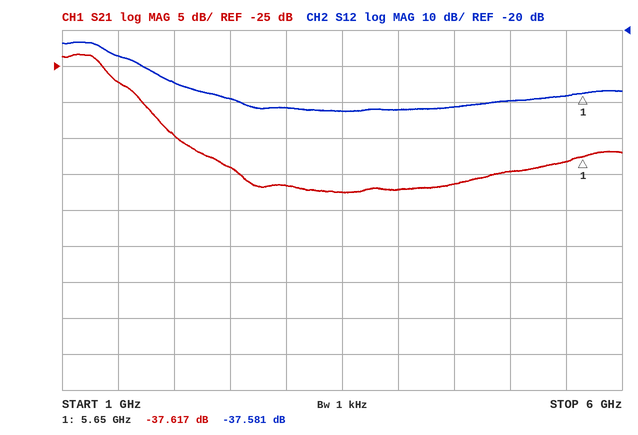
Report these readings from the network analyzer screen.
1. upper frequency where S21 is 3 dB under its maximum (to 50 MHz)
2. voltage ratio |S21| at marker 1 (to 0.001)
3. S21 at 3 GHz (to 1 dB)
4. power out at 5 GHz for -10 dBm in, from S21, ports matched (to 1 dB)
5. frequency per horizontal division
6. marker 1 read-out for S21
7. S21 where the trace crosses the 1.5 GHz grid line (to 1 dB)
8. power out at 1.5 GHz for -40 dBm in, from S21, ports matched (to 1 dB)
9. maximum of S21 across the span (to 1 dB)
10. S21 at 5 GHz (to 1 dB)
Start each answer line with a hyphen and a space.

- 1.45 GHz
- 0.013
- -42 dB
- -50 dBm
- 500 MHz
- -37.617 dB
- -27 dB
- -67 dBm
- -23 dB
- -40 dB
